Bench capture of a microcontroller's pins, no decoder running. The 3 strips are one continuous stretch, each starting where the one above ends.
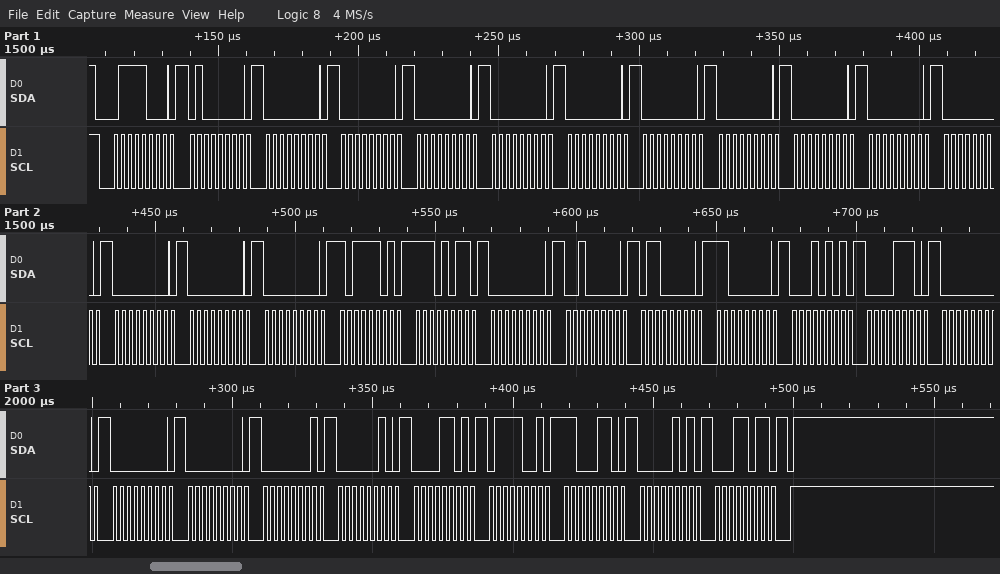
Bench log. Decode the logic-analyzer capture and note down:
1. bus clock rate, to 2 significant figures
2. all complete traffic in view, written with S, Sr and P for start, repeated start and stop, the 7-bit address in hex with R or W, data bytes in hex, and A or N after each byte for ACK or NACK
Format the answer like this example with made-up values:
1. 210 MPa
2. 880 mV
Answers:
1. 400 kHz
2. S 3CW A 40 A 00 A 00 A 00 A 00 A 00 A 00 A 00 A 00 A 00 A 00 A 00 A 00 A 00 A BD A EB A 00 A 20 A 60 A C0 A 15 A 0E A 00 A 00 A 00 A 01 A 02 A 0D A 79 A C6 A 05 A 1B A P
